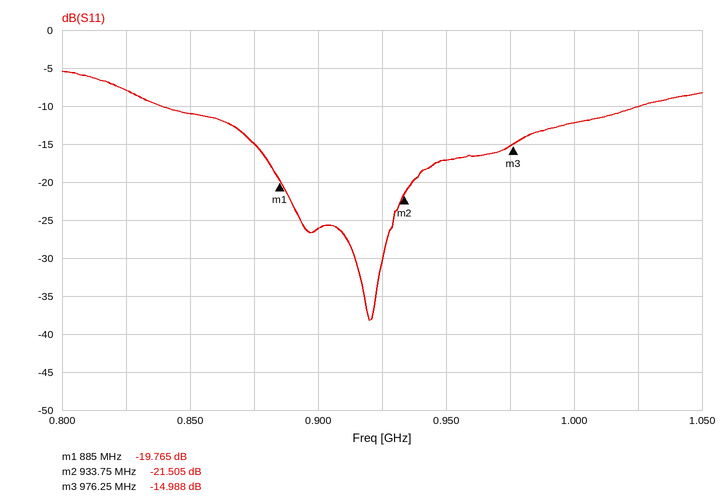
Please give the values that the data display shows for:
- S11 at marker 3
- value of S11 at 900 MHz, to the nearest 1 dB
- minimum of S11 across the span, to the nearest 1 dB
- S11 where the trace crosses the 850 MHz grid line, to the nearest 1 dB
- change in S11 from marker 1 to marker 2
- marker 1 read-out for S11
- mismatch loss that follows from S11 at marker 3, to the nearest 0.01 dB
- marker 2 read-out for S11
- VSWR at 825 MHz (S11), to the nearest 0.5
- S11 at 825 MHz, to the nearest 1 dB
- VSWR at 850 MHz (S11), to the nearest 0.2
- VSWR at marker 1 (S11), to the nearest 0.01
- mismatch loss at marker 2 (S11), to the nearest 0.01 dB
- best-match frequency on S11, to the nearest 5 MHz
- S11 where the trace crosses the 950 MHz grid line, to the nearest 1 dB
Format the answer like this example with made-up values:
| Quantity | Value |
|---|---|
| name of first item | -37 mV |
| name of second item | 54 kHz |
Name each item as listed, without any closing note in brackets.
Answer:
| Quantity | Value |
|---|---|
| S11 at marker 3 | -14.988 dB |
| value of S11 at 900 MHz, to the nearest 1 dB | -26 dB |
| minimum of S11 across the span, to the nearest 1 dB | -38 dB |
| S11 where the trace crosses the 850 MHz grid line, to the nearest 1 dB | -11 dB |
| change in S11 from marker 1 to marker 2 | -1.740 dB |
| marker 1 read-out for S11 | -19.765 dB |
| mismatch loss that follows from S11 at marker 3, to the nearest 0.01 dB | 0.14 dB |
| marker 2 read-out for S11 | -21.505 dB |
| VSWR at 825 MHz (S11), to the nearest 0.5 | 2.5 |
| S11 at 825 MHz, to the nearest 1 dB | -8 dB |
| VSWR at 850 MHz (S11), to the nearest 0.2 | 1.8 |
| VSWR at marker 1 (S11), to the nearest 0.01 | 1.23 |
| mismatch loss at marker 2 (S11), to the nearest 0.01 dB | 0.03 dB |
| best-match frequency on S11, to the nearest 5 MHz | 920 MHz |
| S11 where the trace crosses the 950 MHz grid line, to the nearest 1 dB | -17 dB |
